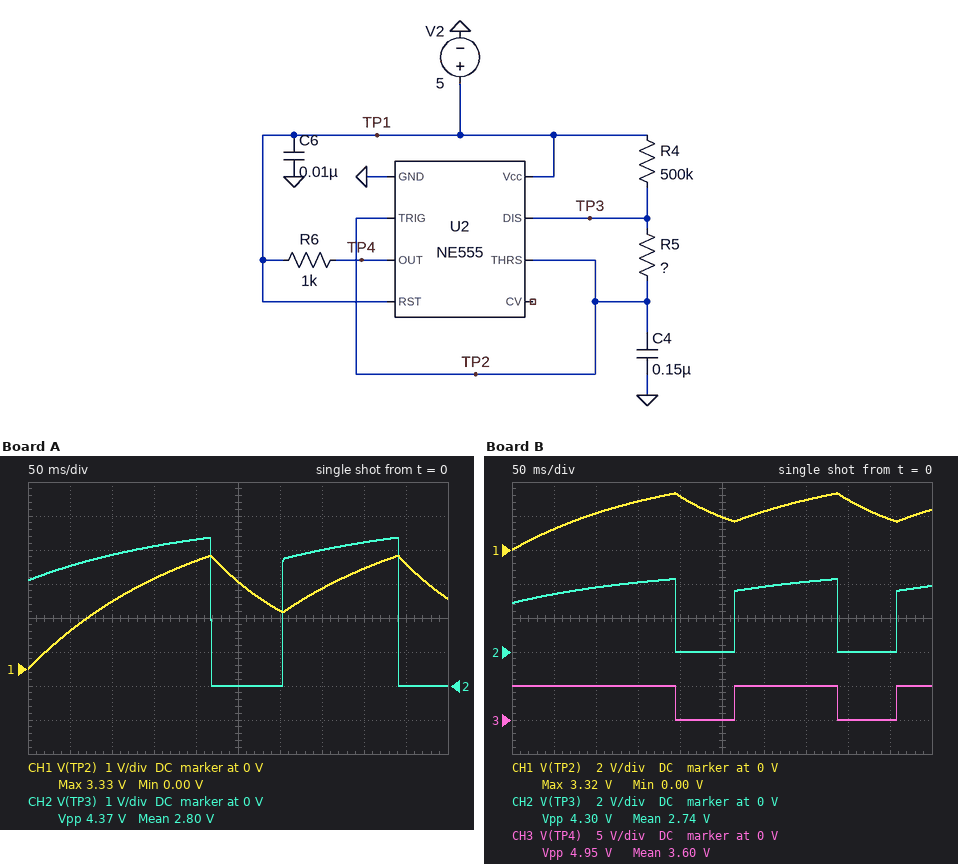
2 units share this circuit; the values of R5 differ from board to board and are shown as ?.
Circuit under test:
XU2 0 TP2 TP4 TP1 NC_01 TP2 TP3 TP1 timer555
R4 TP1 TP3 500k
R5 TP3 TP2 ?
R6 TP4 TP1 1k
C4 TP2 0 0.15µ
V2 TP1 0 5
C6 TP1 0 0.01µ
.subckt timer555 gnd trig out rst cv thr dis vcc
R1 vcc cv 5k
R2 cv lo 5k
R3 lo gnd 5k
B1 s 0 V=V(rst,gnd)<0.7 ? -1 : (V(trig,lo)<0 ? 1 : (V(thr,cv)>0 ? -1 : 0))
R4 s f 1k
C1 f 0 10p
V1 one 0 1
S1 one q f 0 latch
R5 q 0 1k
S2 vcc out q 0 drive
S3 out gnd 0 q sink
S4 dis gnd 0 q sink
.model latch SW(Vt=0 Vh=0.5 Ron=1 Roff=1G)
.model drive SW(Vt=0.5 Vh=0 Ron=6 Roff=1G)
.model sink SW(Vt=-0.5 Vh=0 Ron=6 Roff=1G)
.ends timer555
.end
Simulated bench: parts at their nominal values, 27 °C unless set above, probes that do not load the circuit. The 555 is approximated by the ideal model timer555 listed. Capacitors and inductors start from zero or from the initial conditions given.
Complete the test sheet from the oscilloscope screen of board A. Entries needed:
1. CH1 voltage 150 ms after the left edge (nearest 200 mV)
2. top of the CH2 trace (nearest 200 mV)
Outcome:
2.6 V
4.4 V
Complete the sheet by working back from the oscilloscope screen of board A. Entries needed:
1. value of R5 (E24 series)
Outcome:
820 kΩ
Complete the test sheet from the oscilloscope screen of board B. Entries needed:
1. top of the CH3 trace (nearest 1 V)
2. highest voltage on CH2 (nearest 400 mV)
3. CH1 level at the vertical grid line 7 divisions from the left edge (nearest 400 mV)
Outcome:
5 V
4.4 V
2.8 V
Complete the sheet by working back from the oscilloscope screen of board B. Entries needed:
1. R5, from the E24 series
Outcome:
680 kΩ
